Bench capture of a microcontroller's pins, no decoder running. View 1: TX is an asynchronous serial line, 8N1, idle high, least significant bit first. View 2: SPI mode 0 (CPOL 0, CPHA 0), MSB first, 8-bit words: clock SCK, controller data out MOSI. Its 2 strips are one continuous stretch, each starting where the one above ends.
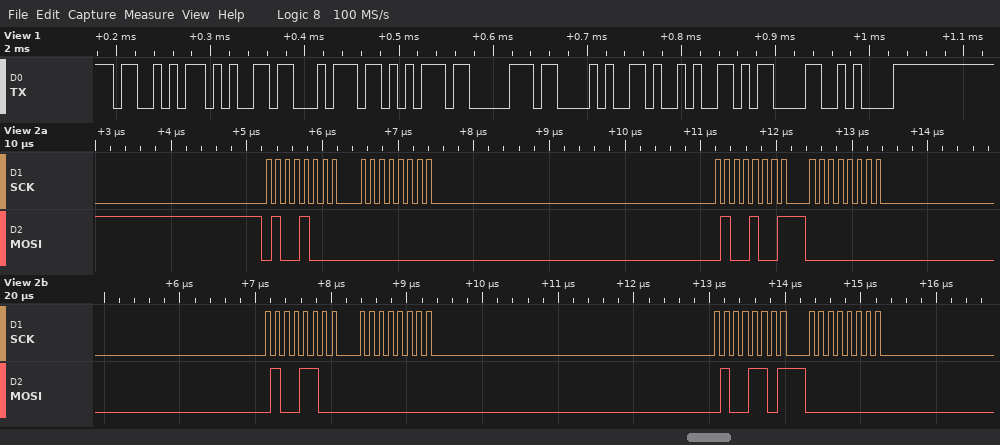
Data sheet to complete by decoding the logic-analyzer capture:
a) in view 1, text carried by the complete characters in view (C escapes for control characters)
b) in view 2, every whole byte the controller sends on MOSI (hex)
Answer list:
"Setup()\r\n"
48 00 49 00 4C 00 4D 00
